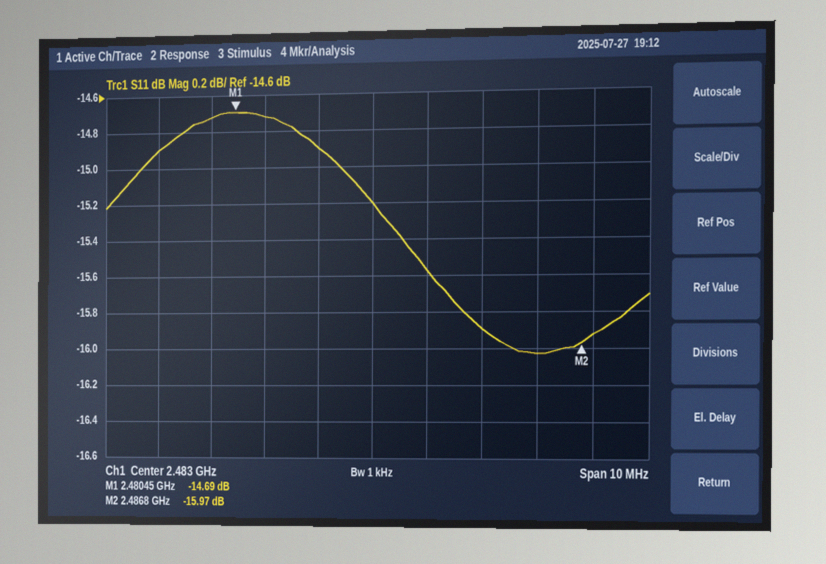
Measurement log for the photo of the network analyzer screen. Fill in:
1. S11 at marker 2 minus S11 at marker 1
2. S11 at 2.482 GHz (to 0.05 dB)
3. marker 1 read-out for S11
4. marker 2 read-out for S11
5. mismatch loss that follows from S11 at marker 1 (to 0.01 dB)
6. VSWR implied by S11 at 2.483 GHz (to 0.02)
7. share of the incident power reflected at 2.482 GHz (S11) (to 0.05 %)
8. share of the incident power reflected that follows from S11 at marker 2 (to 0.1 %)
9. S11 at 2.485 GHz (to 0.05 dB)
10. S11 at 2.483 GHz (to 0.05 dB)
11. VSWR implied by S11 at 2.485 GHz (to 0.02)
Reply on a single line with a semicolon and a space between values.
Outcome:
-1.28 dB; -14.90 dB; -14.69 dB; -15.97 dB; 0.15 dB; 1.42; 3.25 %; 2.5 %; -15.90 dB; -15.20 dB; 1.38
